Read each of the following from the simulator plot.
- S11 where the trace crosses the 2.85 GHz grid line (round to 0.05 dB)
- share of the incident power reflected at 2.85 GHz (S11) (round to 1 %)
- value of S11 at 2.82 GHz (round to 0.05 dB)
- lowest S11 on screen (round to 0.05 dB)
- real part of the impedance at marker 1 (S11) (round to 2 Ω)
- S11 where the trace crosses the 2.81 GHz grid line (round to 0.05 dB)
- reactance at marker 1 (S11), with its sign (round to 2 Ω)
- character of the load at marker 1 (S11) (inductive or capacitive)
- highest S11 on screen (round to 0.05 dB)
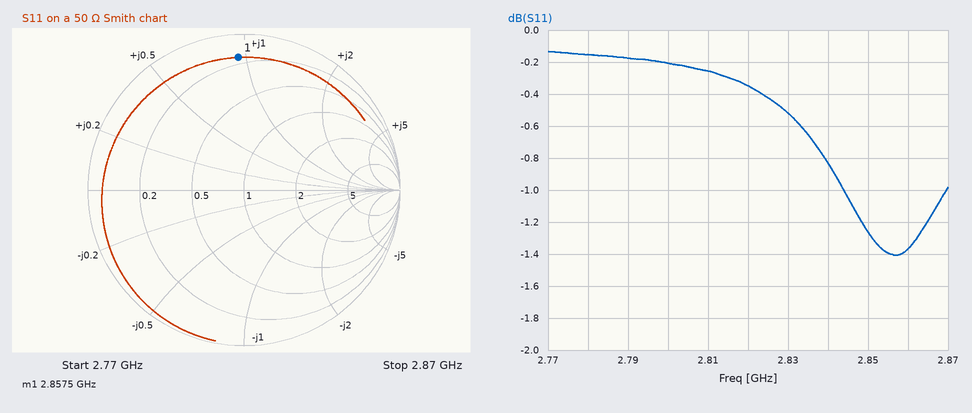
-1.25 dB
75 %
-0.35 dB
-1.40 dB
8 Ω
-0.25 dB
+48 Ω
inductive
-0.15 dB
